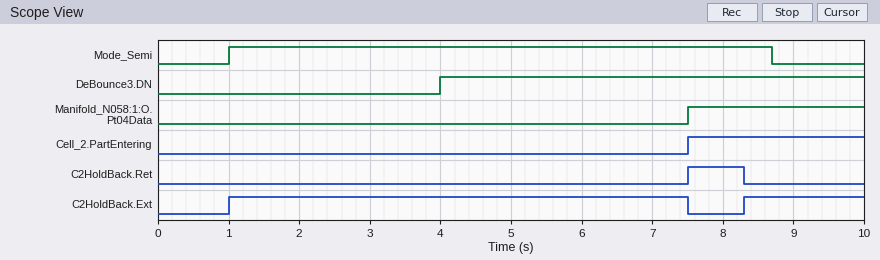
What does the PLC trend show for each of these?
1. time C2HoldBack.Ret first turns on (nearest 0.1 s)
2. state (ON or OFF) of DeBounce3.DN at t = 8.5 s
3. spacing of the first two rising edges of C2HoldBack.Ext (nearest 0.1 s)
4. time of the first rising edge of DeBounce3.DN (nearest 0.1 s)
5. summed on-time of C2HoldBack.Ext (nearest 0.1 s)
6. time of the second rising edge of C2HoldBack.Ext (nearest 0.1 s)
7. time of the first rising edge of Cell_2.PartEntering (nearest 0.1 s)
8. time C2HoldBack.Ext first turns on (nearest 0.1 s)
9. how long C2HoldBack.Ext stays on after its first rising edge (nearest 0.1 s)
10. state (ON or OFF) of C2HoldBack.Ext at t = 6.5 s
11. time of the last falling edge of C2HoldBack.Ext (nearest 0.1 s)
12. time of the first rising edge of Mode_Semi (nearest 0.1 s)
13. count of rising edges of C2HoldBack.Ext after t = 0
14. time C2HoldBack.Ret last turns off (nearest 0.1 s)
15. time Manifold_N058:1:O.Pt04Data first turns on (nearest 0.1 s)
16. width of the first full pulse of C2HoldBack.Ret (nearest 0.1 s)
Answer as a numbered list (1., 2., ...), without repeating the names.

1. 7.5 s
2. ON
3. 7.3 s
4. 4.0 s
5. 8.2 s
6. 8.3 s
7. 7.5 s
8. 1.0 s
9. 6.5 s
10. ON
11. 7.5 s
12. 1.0 s
13. 2
14. 8.3 s
15. 7.5 s
16. 0.8 s
